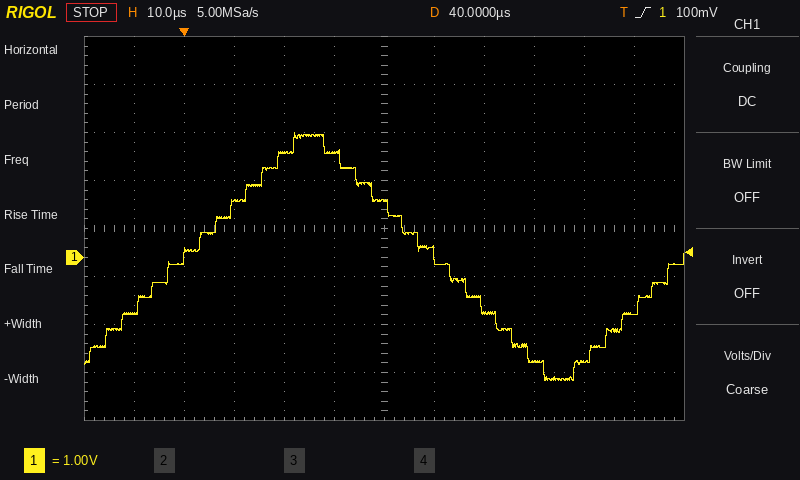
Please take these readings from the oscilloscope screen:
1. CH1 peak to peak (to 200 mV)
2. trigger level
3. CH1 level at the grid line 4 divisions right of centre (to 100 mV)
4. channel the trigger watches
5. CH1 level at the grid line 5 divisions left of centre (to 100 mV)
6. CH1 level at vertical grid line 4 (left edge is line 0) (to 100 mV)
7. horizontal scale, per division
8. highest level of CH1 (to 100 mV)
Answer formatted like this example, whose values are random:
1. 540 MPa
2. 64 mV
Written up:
1. 5.2 V
2. 100 mV
3. -2.2 V
4. CH1
5. -1.2 V
6. 2.2 V
7. 10 µs
8. 2.6 V
